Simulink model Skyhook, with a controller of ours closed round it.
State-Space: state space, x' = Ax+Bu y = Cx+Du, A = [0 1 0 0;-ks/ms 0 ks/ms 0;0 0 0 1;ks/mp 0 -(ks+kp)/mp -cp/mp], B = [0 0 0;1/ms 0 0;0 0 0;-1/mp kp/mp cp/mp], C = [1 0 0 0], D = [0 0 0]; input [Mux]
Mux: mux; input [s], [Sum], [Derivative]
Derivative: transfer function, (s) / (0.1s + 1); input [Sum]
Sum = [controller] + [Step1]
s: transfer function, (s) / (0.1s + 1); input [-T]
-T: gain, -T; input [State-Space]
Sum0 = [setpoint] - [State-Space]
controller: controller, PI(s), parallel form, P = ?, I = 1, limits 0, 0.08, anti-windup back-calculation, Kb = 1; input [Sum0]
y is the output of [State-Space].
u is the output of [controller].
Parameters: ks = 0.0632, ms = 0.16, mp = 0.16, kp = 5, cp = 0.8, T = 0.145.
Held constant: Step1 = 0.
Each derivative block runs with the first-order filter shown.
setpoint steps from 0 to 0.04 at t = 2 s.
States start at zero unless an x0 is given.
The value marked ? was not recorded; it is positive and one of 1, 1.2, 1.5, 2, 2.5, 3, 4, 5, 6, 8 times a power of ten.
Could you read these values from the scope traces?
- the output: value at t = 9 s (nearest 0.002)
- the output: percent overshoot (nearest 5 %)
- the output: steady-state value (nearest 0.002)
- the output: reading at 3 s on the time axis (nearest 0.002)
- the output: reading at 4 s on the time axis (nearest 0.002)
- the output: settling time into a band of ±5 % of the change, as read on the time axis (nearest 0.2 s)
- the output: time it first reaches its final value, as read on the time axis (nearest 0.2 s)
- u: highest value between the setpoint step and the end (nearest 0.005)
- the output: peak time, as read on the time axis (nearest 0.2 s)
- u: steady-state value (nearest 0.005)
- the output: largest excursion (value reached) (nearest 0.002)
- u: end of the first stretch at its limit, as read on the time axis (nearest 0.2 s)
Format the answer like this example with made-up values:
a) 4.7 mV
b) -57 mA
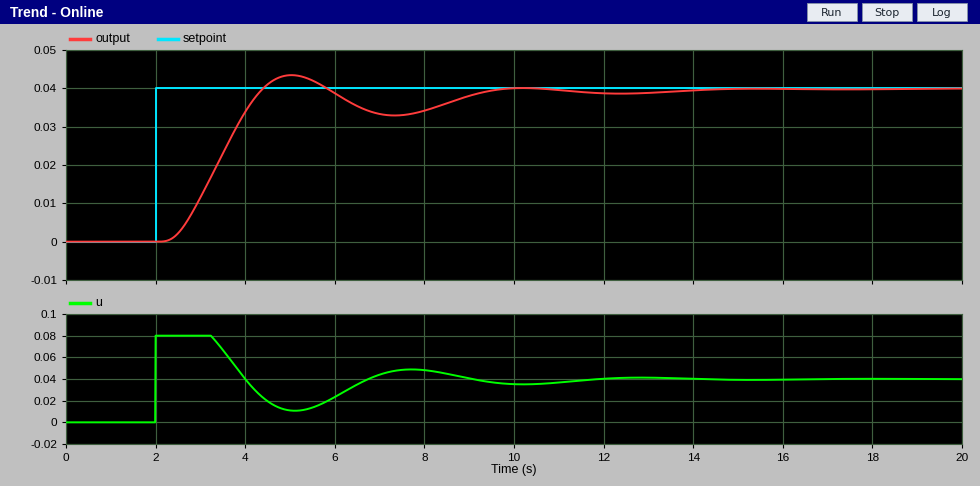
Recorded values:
a) 0.038
b) 10 %
c) 0.040
d) 0.012
e) 0.034
f) 9.0 s
g) 4.4 s
h) 0.080
i) 5.0 s
j) 0.040
k) 0.044
l) 3.2 s
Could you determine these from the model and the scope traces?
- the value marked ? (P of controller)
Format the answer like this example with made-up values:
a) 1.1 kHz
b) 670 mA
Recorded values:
a) 3
